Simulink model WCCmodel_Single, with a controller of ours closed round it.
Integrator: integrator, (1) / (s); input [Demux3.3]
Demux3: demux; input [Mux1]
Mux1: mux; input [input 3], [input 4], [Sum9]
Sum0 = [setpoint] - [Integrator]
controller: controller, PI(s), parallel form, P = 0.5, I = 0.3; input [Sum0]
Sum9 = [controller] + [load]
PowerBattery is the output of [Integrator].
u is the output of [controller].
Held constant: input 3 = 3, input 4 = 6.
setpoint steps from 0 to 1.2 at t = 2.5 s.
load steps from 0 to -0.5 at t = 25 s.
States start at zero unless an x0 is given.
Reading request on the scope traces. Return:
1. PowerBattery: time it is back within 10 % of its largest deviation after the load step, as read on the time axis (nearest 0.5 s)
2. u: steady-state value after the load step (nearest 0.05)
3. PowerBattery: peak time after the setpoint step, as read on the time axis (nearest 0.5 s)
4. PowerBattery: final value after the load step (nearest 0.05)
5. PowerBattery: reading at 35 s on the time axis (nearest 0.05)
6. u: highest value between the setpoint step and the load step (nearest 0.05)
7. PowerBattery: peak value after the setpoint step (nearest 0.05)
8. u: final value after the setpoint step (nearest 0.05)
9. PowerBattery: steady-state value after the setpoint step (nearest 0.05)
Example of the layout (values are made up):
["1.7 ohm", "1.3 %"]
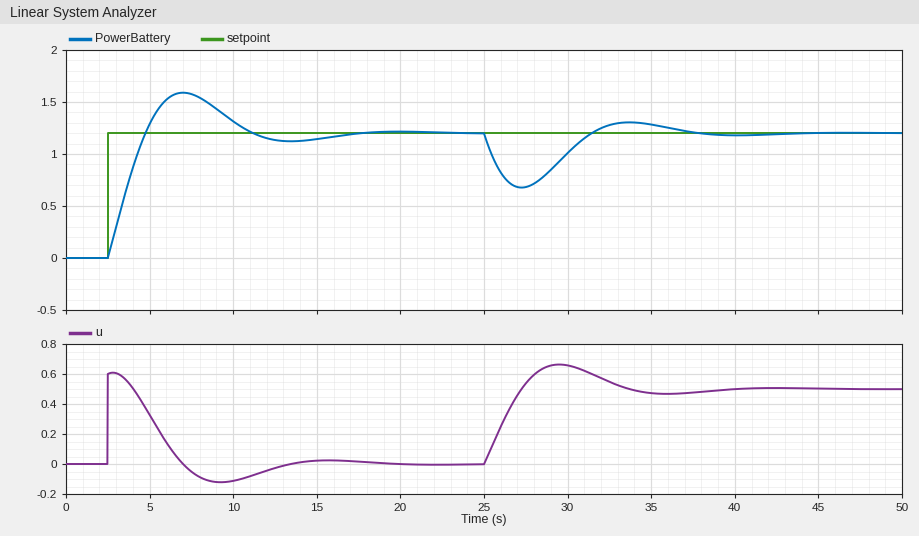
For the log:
["36.0 s", "0.50", "7.0 s", "1.20", "1.30", "0.60", "1.60", "0.00", "1.20"]
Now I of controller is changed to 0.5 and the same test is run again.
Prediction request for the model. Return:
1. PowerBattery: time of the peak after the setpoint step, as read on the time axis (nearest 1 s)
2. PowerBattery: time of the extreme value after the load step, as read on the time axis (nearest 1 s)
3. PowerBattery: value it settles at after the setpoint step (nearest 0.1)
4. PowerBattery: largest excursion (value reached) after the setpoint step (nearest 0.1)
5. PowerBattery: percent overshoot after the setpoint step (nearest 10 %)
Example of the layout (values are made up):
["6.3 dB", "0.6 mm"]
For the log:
["6 s", "27 s", "1.2", "1.7", "40 %"]
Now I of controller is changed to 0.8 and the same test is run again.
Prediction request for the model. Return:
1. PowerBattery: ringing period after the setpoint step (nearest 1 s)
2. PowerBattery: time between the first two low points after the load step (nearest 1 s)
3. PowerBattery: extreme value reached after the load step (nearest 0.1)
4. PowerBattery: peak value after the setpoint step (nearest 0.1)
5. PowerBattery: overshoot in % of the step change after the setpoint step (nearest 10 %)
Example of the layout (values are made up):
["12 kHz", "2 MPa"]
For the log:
["7 s", "7 s", "0.8", "1.8", "50 %"]
